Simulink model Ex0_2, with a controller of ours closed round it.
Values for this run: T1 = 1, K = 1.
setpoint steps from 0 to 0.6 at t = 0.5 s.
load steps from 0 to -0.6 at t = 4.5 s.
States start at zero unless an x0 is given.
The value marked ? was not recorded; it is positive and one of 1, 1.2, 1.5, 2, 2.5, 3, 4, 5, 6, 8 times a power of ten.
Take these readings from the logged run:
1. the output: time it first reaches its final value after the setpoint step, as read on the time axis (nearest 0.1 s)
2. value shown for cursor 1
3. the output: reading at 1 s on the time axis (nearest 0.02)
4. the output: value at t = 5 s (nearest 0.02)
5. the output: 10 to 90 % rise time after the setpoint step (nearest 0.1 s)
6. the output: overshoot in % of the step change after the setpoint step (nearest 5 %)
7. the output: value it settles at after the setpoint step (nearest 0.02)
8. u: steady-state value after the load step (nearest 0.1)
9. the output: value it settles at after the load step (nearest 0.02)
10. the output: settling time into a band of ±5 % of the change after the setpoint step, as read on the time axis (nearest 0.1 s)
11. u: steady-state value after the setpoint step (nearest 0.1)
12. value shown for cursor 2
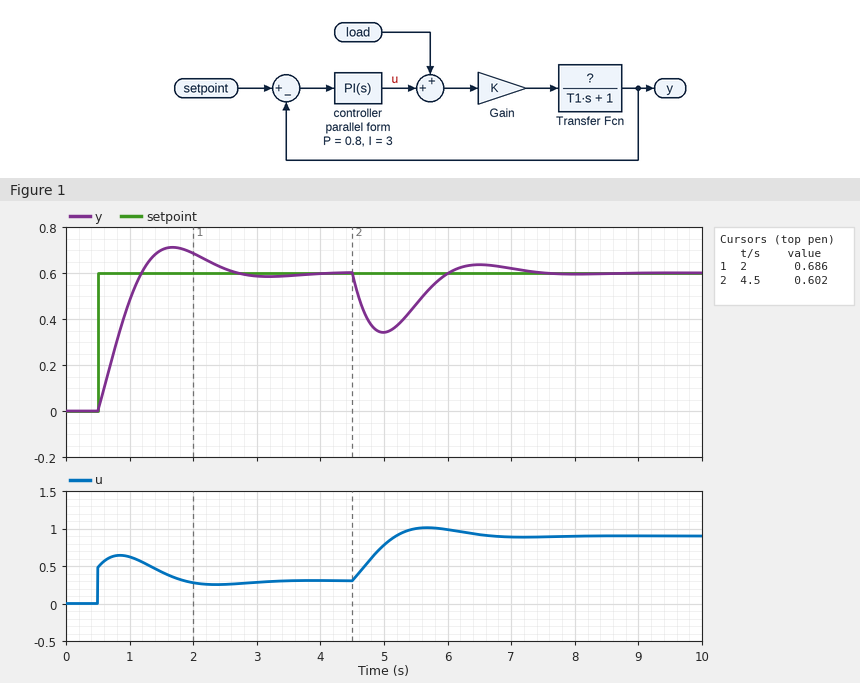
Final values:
1.2 s
0.686
0.48
0.34
0.5 s
20 %
0.60
0.9
0.60
2.4 s
0.3
0.602
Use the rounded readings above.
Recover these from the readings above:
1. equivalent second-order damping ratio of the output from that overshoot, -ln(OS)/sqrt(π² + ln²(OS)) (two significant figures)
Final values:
0.46
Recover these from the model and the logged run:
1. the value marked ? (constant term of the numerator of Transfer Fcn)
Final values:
2
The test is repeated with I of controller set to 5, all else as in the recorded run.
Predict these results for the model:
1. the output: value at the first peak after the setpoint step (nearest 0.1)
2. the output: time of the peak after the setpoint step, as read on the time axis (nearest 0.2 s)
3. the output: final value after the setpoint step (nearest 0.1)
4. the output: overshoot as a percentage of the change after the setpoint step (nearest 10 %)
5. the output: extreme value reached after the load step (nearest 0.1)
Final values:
0.8
1.4 s
0.6
30 %
0.4
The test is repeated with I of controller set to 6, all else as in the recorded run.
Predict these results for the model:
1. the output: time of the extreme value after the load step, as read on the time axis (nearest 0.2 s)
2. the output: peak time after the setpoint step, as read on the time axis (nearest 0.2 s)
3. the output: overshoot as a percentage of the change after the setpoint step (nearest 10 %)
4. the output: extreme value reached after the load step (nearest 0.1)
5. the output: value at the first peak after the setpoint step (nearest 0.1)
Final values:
4.8 s
1.4 s
30 %
0.4
0.8
